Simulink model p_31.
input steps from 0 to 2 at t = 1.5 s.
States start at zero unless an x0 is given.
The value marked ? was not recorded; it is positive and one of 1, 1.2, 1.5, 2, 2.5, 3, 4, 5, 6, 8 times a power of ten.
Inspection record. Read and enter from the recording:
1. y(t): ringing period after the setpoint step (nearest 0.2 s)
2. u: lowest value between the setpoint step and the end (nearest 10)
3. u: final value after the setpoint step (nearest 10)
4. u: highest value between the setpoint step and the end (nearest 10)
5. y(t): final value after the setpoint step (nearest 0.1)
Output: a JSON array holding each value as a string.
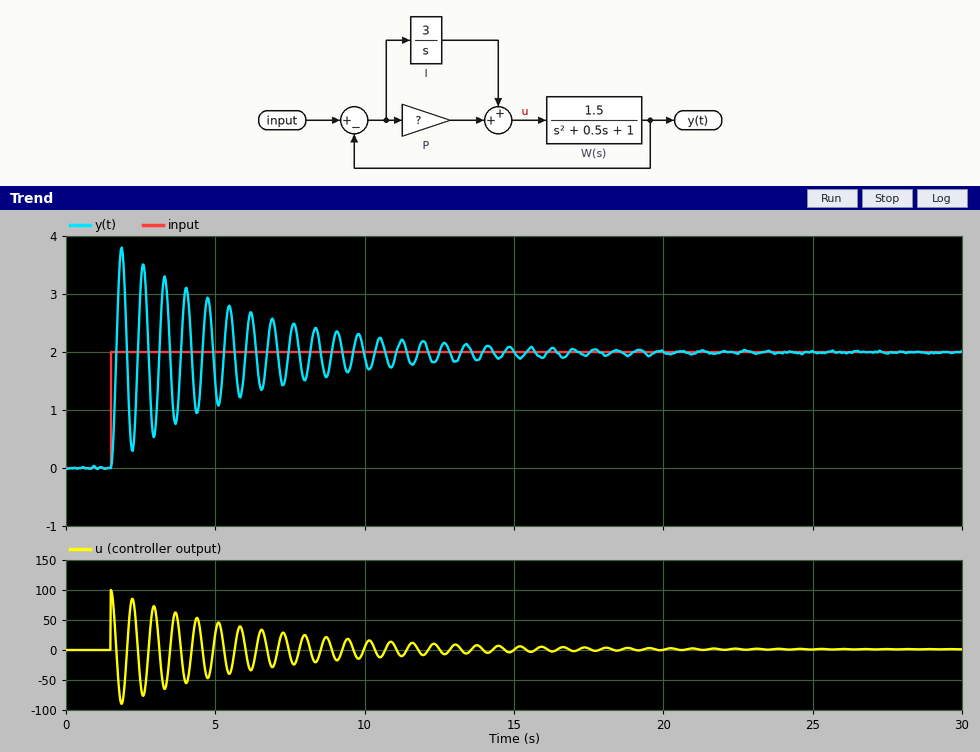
["0.8 s", "-90", "0", "100", "2.0"]
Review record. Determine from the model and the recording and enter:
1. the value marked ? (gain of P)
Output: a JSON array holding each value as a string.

["50"]
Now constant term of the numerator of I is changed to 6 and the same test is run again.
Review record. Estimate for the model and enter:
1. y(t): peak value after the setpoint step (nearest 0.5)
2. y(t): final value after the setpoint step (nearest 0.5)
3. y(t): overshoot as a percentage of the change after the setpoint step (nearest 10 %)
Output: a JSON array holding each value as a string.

["4.0", "2.0", "90 %"]
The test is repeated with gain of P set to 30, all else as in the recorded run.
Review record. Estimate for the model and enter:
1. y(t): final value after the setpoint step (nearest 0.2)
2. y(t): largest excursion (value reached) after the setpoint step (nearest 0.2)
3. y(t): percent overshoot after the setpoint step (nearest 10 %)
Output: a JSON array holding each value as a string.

["2.0", "3.8", "90 %"]
